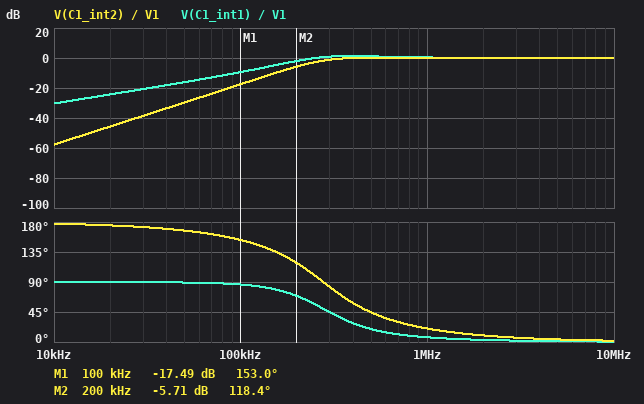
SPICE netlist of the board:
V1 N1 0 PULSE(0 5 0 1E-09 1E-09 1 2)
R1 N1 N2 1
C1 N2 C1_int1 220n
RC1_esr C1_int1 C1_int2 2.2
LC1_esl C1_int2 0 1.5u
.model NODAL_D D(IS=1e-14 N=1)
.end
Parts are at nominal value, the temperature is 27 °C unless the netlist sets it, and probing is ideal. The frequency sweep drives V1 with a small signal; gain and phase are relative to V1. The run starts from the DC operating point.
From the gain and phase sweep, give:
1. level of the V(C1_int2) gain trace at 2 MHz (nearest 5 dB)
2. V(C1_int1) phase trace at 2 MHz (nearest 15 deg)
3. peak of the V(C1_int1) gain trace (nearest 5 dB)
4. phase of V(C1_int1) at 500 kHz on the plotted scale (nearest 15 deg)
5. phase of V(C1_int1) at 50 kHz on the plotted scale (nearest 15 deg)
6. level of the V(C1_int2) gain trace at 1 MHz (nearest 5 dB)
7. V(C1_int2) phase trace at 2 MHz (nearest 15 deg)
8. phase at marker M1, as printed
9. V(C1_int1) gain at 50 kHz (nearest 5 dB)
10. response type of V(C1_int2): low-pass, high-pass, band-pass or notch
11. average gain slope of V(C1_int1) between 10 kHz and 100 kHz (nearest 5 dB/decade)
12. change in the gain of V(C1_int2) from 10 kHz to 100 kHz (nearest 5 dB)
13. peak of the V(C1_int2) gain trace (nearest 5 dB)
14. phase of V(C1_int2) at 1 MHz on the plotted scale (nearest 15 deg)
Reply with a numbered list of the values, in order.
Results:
1. 0 dB
2. 0 deg
3. 0 dB
4. 15 deg
5. 90 deg
6. 0 dB
7. 15 deg
8. 153.0 deg
9. -15 dB
10. high-pass
11. 20 dB/decade
12. 40 dB
13. 0 dB
14. 15 deg
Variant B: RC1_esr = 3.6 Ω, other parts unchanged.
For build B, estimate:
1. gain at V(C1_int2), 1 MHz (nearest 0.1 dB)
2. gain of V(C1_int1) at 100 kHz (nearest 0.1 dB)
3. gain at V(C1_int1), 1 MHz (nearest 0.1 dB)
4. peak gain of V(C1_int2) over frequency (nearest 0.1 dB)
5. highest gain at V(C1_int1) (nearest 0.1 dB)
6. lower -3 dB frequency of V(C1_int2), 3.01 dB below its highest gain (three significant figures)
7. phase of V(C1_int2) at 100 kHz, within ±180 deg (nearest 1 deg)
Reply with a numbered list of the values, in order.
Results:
1. -0.4 dB
2. -6.4 dB
3. 0.2 dB
4. 0 dB
5. 0.4 dB
6. 361 kHz
7. 144 deg
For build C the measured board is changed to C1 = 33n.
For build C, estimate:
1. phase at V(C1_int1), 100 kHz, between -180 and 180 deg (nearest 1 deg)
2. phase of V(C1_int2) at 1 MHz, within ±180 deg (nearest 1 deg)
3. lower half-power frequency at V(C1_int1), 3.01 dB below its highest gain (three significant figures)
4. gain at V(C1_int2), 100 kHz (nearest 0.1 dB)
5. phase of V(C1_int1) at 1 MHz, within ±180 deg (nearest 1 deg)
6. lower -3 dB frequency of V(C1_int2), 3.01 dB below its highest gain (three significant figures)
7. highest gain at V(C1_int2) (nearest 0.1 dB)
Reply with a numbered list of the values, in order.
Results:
1. 109 deg
2. 35 deg
3. 611 kHz
4. -34.0 dB
5. 22 deg
6. 616 kHz
7. 6.7 dB
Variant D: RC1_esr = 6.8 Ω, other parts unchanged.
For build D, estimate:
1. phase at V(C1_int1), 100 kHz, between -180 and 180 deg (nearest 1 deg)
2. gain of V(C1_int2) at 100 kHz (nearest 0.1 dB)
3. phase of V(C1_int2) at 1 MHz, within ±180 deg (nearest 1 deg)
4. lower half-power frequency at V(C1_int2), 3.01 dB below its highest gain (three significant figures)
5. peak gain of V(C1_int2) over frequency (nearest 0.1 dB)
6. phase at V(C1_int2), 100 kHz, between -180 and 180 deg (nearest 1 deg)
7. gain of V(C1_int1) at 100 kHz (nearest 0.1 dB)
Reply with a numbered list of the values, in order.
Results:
1. 47 deg
2. -20.5 dB
3. 42 deg
4. 736 kHz
5. 0 dB
6. 129 deg
7. -3.3 dB
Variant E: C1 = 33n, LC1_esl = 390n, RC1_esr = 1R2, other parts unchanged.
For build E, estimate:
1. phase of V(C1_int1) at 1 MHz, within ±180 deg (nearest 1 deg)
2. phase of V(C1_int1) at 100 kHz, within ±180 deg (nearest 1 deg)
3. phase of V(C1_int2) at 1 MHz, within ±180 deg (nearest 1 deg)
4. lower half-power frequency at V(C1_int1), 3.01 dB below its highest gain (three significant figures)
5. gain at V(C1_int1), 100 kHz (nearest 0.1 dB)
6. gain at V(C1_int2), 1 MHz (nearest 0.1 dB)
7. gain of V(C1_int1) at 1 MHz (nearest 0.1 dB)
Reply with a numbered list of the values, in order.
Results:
1. 111 deg
2. 99 deg
3. 137 deg
4. 1.17 MHz
5. -31.9 dB
6. -2.4 dB
7. -1.5 dB
